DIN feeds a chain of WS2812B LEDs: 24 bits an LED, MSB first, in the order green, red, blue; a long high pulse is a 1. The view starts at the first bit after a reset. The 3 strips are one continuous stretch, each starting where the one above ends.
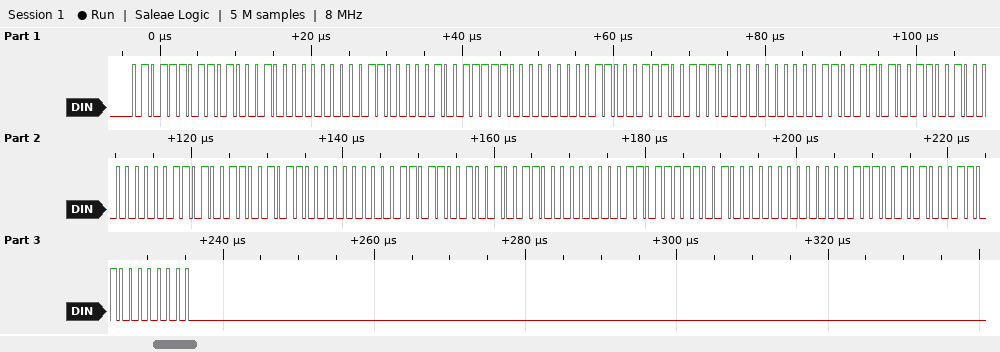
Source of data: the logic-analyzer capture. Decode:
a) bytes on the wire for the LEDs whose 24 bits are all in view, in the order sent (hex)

5D A2 00 60 9F 00 63 9C 00 66 99 00 69 96 00 6C 93 00 6F 90 00 72 8D 00
